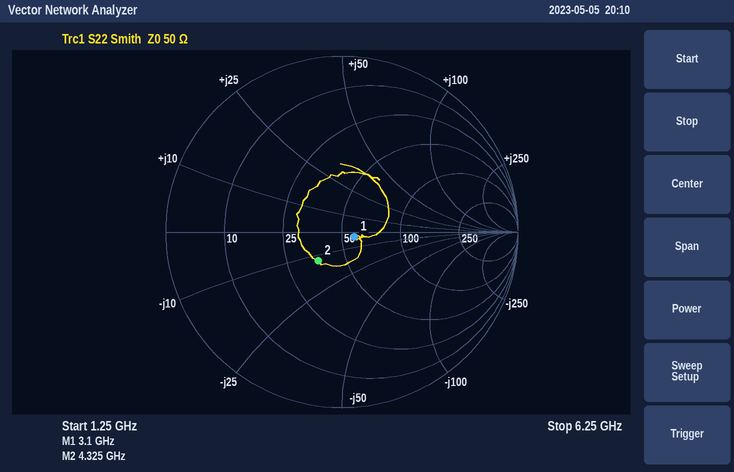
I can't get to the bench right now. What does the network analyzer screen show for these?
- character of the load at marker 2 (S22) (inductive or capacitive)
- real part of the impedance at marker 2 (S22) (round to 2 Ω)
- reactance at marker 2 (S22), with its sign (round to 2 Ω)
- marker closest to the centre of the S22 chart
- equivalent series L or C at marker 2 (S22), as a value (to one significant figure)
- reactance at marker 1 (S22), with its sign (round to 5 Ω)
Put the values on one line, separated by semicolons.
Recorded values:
capacitive; 36 Ω; -12 Ω; marker 1; 3 pF; -5 Ω
